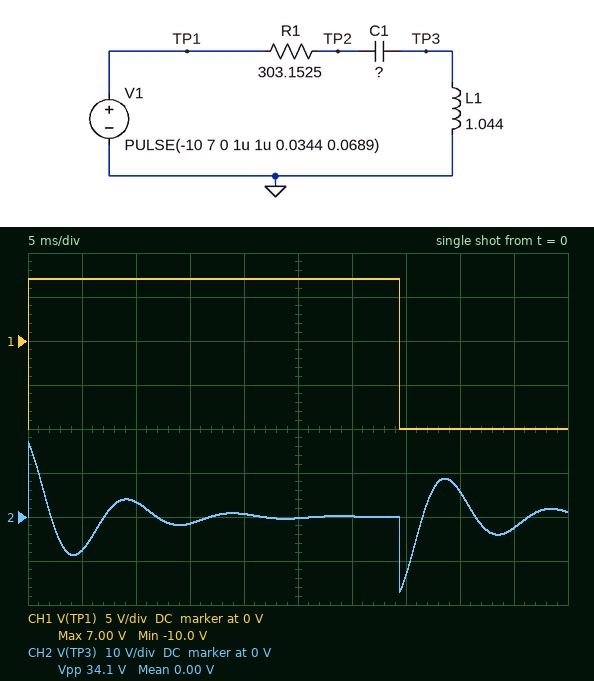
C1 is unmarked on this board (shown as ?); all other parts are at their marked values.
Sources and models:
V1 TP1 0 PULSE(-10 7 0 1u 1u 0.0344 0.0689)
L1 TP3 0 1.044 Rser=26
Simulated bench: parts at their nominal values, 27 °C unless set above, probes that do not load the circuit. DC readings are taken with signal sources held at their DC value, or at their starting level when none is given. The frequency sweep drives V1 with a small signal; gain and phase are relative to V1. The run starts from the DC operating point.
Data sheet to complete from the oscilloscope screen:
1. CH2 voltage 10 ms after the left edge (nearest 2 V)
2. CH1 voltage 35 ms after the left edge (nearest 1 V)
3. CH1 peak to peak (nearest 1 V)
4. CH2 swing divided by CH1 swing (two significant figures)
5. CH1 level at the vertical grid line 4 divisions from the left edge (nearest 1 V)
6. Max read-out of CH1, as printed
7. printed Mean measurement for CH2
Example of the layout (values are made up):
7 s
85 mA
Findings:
4 V
-10 V
17 V
2.0
7 V
7.00 V
0.00 V
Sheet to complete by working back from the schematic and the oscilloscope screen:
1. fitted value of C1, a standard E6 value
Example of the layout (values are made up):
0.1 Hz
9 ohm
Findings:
2.2 µF
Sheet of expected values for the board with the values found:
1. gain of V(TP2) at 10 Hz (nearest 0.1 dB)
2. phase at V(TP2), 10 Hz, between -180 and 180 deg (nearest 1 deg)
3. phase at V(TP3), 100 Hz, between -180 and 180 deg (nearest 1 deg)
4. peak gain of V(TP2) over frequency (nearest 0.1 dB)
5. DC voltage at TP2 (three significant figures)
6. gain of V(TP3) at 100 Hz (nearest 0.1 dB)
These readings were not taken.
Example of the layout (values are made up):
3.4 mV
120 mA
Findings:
0 dB
-2 deg
99 deg
0 dB
-10.0 V
5.8 dB
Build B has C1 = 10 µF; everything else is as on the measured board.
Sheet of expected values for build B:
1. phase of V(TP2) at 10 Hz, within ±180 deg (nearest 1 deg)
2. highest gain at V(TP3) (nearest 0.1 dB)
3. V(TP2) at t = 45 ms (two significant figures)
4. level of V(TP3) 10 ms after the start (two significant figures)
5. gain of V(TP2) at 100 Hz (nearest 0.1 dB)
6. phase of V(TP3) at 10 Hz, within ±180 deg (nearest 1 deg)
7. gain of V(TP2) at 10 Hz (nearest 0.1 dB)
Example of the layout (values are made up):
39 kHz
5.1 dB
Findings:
-11 deg
1.2 dB
-8.9 V
-3.9 V
-1.6 dB
146 deg
-0.2 dB
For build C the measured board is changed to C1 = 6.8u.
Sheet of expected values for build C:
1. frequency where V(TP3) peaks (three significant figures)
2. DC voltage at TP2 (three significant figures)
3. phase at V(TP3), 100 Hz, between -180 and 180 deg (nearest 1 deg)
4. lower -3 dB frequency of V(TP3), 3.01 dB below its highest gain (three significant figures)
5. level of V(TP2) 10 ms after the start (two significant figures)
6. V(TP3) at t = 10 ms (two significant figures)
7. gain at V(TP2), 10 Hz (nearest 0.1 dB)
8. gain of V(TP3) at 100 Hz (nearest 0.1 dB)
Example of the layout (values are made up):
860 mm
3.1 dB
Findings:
74.2 Hz
-10.0 V
36 deg
50.3 Hz
7.8 V
-3.0 V
-0.1 dB
1.8 dB
